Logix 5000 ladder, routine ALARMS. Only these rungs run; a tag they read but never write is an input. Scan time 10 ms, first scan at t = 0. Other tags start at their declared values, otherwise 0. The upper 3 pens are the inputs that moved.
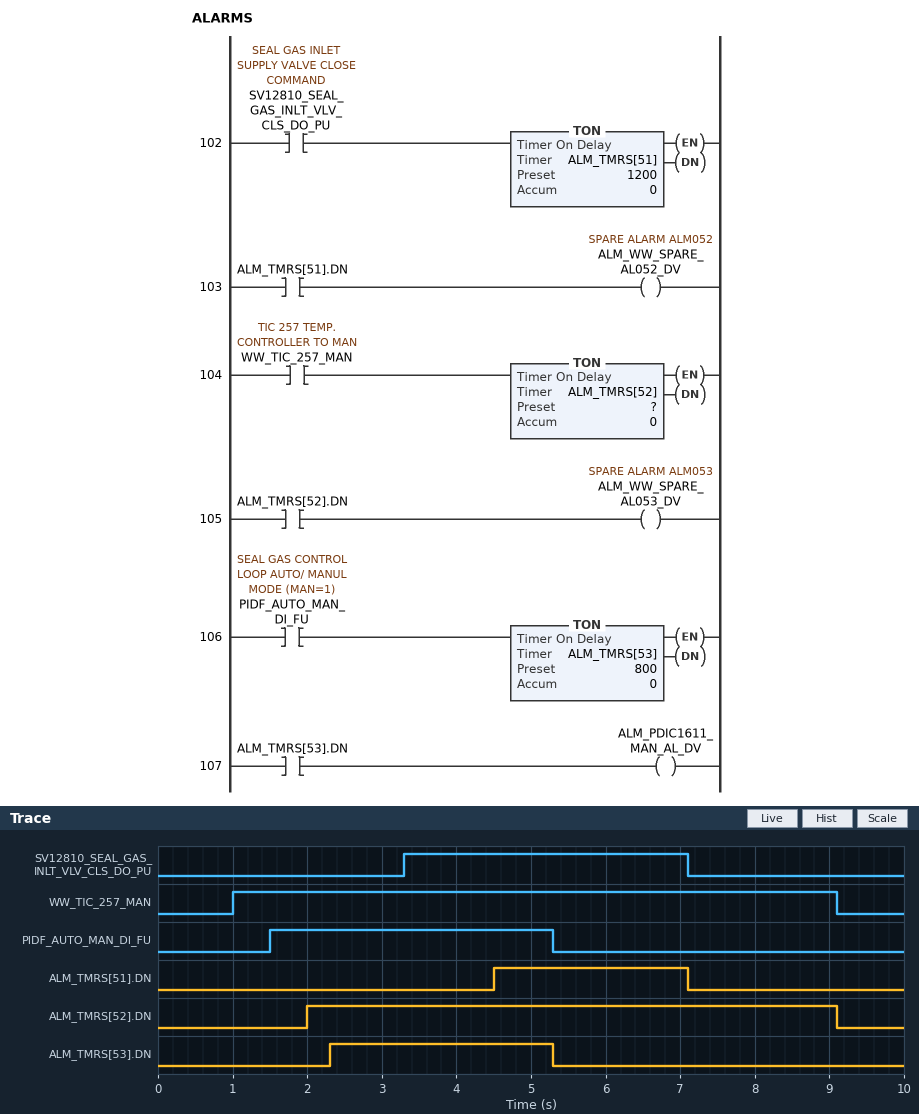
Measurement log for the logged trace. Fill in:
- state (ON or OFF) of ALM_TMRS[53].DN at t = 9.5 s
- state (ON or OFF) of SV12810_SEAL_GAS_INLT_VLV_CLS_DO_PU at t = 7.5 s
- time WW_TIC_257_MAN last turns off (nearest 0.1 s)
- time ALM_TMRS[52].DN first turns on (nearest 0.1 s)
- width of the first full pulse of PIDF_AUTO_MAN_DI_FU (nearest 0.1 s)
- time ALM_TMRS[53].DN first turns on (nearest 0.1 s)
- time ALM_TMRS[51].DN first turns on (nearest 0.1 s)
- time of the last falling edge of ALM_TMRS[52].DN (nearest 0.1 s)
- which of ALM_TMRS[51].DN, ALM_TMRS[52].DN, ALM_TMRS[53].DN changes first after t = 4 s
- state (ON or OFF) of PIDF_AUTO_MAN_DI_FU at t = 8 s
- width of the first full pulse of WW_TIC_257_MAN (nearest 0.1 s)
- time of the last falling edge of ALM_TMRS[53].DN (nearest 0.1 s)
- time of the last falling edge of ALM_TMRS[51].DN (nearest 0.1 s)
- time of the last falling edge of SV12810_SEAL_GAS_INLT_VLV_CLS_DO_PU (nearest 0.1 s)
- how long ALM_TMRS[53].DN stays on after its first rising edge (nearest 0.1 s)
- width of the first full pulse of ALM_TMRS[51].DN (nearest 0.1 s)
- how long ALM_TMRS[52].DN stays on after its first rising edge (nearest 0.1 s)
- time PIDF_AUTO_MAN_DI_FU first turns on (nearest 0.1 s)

OFF
OFF
9.1 s
2.0 s
3.8 s
2.3 s
4.5 s
9.1 s
ALM_TMRS[51].DN
OFF
8.1 s
5.3 s
7.1 s
7.1 s
3.0 s
2.6 s
7.1 s
1.5 s
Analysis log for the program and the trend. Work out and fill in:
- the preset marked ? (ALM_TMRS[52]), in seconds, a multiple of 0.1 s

1.0 s
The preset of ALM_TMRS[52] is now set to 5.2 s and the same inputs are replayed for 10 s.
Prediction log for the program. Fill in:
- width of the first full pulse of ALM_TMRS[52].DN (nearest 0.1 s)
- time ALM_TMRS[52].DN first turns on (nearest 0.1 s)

2.9 s
6.2 s
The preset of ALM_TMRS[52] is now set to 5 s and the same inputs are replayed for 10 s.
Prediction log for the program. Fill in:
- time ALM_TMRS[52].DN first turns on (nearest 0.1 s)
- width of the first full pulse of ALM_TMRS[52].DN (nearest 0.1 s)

6.0 s
3.1 s
